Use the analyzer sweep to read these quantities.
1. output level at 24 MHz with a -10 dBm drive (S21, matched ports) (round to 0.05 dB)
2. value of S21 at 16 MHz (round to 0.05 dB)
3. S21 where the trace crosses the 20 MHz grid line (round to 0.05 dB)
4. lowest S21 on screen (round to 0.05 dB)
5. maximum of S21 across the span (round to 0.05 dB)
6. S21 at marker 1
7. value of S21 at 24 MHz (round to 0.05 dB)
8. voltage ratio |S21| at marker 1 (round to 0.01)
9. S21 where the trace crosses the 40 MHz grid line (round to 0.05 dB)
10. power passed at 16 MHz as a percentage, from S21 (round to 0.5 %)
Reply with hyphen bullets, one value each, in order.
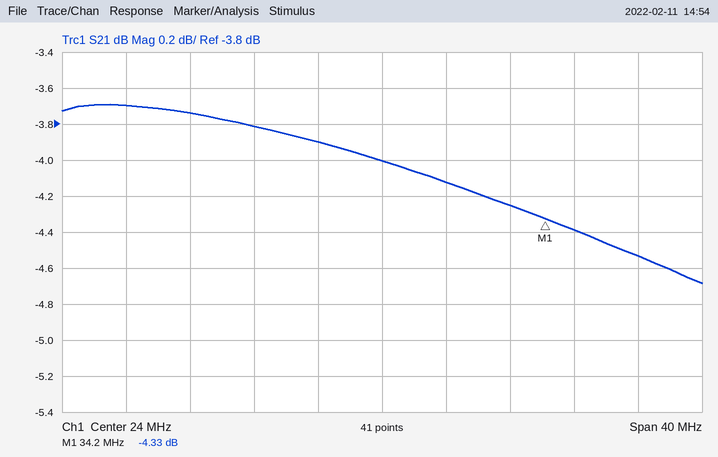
- -14.00 dBm
- -3.80 dB
- -3.90 dB
- -4.70 dB
- -3.70 dB
- -4.33 dB
- -4.00 dB
- 0.61
- -4.55 dB
- 41.5 %
